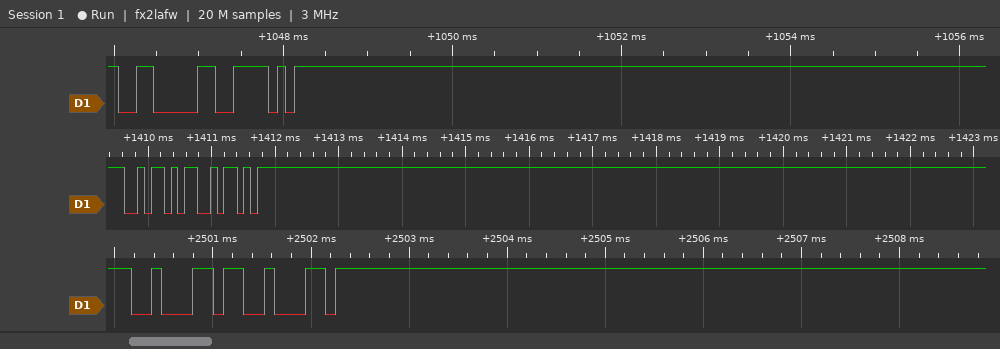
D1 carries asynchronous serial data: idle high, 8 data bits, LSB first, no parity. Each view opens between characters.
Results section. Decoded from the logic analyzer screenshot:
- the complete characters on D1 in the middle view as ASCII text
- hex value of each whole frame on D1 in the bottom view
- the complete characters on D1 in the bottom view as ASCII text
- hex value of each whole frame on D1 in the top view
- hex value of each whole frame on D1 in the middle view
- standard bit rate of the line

"ZZ"
62, 62
"bb"
06, 5E
5A, 5A
9600 baud
